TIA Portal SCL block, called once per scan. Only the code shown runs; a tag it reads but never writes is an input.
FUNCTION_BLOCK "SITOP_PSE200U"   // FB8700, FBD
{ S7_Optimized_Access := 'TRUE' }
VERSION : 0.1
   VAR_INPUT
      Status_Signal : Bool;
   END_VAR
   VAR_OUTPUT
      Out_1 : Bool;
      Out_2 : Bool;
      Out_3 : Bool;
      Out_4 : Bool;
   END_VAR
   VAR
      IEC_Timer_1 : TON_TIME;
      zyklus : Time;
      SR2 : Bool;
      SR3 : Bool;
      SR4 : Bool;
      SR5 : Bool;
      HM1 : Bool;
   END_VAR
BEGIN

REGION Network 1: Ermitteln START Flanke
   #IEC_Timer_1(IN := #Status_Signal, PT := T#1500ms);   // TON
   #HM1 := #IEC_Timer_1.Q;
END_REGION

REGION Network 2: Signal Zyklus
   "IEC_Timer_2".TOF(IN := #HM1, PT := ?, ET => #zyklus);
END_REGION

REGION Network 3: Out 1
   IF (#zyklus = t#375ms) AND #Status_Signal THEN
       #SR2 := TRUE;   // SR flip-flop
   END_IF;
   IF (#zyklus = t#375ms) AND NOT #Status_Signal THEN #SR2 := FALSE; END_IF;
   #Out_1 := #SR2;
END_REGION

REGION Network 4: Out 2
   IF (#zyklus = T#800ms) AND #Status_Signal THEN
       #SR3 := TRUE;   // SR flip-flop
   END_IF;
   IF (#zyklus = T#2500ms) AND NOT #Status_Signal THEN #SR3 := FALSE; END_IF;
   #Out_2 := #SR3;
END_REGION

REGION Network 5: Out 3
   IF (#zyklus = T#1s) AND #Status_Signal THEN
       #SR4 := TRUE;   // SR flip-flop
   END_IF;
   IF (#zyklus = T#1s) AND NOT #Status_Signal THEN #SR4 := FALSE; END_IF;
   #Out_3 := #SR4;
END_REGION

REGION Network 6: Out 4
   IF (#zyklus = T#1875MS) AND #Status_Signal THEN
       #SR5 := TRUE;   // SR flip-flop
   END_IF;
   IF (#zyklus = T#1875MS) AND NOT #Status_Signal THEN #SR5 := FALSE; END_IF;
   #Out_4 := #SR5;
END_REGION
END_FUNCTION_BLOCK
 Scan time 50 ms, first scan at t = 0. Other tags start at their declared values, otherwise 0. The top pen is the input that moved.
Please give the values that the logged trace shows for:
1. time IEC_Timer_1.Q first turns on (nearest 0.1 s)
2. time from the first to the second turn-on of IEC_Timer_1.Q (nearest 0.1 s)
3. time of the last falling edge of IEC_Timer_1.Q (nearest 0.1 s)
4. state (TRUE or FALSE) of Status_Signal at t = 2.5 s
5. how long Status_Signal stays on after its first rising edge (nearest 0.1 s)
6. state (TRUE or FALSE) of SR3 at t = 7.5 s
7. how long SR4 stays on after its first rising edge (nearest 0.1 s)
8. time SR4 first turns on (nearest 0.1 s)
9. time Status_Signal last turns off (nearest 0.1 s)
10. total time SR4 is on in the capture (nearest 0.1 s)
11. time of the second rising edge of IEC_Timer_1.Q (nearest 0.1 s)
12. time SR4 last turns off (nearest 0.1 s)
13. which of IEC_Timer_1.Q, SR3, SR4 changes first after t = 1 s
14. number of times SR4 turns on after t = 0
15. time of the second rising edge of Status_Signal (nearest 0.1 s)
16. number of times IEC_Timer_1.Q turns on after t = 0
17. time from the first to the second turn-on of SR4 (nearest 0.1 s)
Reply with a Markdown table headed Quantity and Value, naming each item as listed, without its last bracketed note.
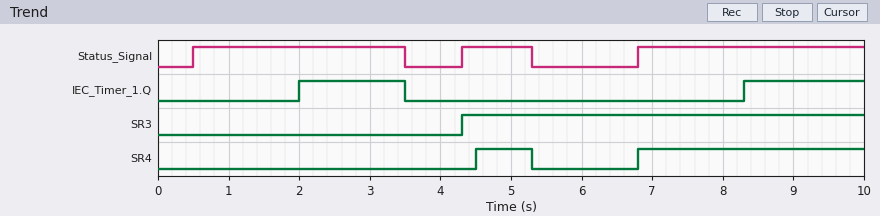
| Quantity | Value |
|---|---|
| time IEC_Timer_1.Q first turns on | 2.0 s |
| time from the first to the second turn-on of IEC_Timer_1.Q | 6.3 s |
| time of the last falling edge of IEC_Timer_1.Q | 3.5 s |
| state (TRUE or FALSE) of Status_Signal at t = 2.5 s | TRUE |
| how long Status_Signal stays on after its first rising edge | 3.0 s |
| state (TRUE or FALSE) of SR3 at t = 7.5 s | TRUE |
| how long SR4 stays on after its first rising edge | 0.8 s |
| time SR4 first turns on | 4.5 s |
| time Status_Signal last turns off | 5.3 s |
| total time SR4 is on in the capture | 4.0 s |
| time of the second rising edge of IEC_Timer_1.Q | 8.3 s |
| time SR4 last turns off | 5.3 s |
| which of IEC_Timer_1.Q, SR3, SR4 changes first after t = 1 s | IEC_Timer_1.Q |
| number of times SR4 turns on after t = 0 | 2 |
| time of the second rising edge of Status_Signal | 4.3 s |
| number of times IEC_Timer_1.Q turns on after t = 0 | 2 |
| time from the first to the second turn-on of SR4 | 2.3 s |
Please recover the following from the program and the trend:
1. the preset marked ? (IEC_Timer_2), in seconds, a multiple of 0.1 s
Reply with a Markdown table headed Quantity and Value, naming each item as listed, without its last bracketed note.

| Quantity | Value |
|---|---|
| the preset marked ? (IEC_Timer_2), in seconds, a multiple of 0.1 s | 1.0 s |
